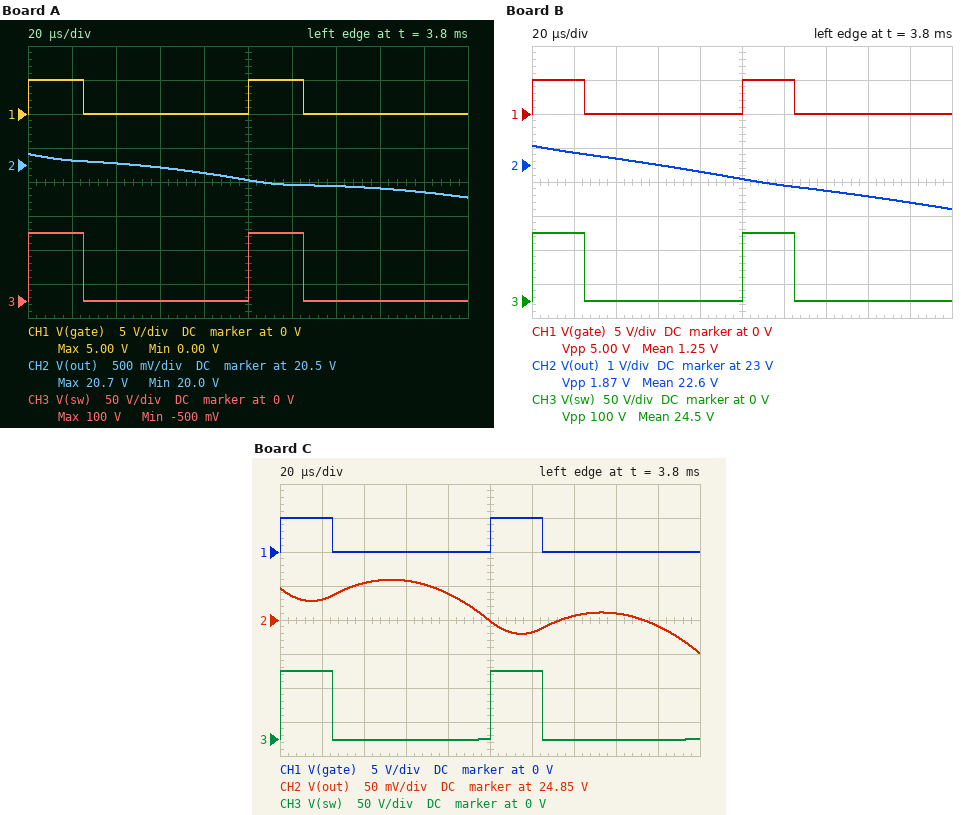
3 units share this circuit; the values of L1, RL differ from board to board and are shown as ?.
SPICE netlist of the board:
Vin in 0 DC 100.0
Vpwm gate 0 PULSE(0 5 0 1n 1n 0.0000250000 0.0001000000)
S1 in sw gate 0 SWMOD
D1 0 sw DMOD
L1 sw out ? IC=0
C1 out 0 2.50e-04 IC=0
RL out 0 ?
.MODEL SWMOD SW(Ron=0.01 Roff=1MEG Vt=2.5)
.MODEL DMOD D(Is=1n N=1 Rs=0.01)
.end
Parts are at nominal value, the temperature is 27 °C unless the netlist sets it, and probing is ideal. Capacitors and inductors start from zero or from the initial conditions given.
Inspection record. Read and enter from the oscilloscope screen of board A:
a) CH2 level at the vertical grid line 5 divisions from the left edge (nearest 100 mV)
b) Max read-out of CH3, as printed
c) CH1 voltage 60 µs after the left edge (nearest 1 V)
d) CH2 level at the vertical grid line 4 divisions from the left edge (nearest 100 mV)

20.3 V
100 V
0 V
20.4 V
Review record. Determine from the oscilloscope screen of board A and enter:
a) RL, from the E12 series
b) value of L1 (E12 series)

8.2 Ω
1.5 mH
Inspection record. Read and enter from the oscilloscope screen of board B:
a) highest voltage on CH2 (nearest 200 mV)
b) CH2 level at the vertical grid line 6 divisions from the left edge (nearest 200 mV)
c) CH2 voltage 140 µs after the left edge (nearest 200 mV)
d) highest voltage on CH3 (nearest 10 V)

23.6 V
22.4 V
22.2 V
100 V
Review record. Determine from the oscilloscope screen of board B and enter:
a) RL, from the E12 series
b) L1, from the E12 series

6.8 Ω
2.2 mH
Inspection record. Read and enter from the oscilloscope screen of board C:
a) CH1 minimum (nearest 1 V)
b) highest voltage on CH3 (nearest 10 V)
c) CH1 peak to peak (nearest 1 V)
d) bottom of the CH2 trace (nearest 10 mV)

0 V
100 V
5 V
24.80 V
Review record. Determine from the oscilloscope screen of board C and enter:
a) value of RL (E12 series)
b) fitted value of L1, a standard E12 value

1.8 Ω
1.8 mH
